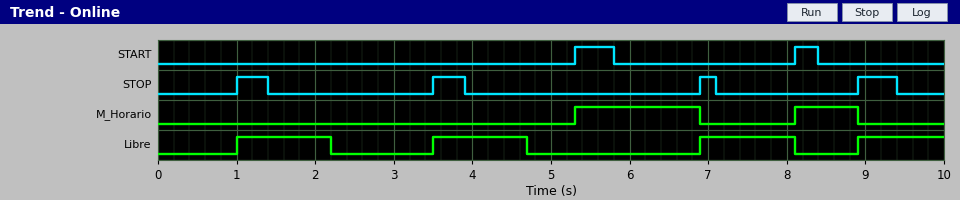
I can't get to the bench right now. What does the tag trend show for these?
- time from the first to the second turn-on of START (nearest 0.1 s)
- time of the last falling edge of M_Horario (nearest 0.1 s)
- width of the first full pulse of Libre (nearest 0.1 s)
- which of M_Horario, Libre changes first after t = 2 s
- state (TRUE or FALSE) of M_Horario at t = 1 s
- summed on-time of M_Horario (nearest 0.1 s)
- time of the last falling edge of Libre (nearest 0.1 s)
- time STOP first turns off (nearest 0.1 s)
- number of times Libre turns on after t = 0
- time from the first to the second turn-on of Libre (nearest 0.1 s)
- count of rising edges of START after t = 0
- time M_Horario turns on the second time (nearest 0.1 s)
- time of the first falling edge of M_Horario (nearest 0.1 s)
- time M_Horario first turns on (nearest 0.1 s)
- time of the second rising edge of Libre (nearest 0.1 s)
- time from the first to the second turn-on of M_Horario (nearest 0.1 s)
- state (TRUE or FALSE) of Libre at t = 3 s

2.8 s
8.9 s
1.2 s
Libre
FALSE
2.4 s
8.1 s
1.4 s
4
2.5 s
2
8.1 s
6.9 s
5.3 s
3.5 s
2.8 s
FALSE
